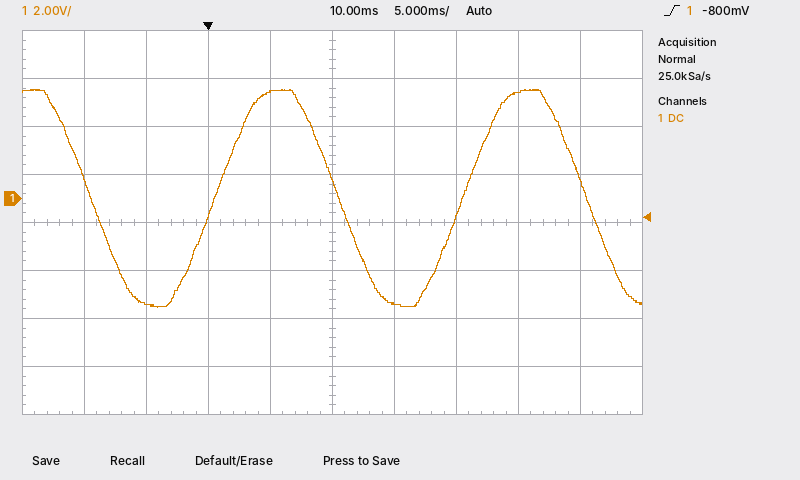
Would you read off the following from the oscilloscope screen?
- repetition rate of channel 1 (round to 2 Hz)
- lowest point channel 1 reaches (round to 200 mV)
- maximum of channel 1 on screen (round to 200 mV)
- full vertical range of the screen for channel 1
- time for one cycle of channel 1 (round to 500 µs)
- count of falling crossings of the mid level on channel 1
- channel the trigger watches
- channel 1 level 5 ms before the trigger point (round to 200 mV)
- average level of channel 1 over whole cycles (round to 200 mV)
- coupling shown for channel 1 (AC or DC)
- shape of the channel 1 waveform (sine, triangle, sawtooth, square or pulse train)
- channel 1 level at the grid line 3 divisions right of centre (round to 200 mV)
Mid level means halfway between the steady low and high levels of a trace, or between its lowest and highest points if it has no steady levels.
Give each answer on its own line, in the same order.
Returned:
50 Hz
-4.6 V
4.6 V
16 V
20.0 ms
3
channel 1
-4.4 V
0.0 V
DC
sine
4.4 V
